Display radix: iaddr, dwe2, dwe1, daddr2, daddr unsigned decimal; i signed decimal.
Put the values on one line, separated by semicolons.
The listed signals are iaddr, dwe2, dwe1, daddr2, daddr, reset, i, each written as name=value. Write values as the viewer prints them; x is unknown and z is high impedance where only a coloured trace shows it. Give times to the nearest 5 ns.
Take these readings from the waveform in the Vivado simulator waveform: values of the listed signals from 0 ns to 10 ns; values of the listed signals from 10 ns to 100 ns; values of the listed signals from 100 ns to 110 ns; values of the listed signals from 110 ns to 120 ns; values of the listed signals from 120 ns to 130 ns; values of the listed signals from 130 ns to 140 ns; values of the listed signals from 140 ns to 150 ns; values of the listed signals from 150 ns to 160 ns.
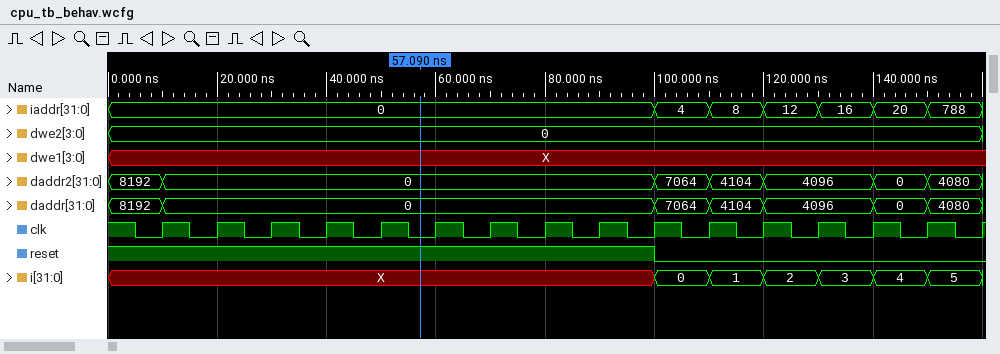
iaddr=0, dwe2=0, dwe1=X, daddr2=8192, daddr=8192, reset=1, i=X; iaddr=0, dwe2=0, dwe1=X, daddr2=0, daddr=0, reset=1, i=X; iaddr=4, dwe2=0, dwe1=X, daddr2=7064, daddr=7064, reset=0, i=0; iaddr=8, dwe2=0, dwe1=X, daddr2=4104, daddr=4104, reset=0, i=1; iaddr=12, dwe2=0, dwe1=X, daddr2=4096, daddr=4096, reset=0, i=2; iaddr=16, dwe2=0, dwe1=X, daddr2=4096, daddr=4096, reset=0, i=3; iaddr=20, dwe2=0, dwe1=X, daddr2=0, daddr=0, reset=0, i=4; iaddr=788, dwe2=0, dwe1=X, daddr2=4080, daddr=4080, reset=0, i=5
